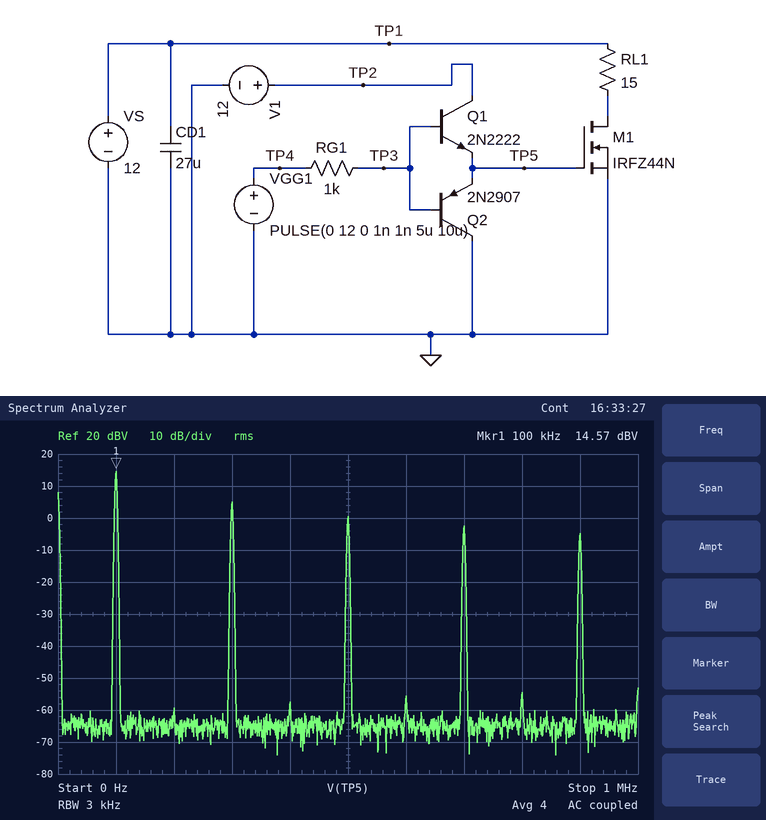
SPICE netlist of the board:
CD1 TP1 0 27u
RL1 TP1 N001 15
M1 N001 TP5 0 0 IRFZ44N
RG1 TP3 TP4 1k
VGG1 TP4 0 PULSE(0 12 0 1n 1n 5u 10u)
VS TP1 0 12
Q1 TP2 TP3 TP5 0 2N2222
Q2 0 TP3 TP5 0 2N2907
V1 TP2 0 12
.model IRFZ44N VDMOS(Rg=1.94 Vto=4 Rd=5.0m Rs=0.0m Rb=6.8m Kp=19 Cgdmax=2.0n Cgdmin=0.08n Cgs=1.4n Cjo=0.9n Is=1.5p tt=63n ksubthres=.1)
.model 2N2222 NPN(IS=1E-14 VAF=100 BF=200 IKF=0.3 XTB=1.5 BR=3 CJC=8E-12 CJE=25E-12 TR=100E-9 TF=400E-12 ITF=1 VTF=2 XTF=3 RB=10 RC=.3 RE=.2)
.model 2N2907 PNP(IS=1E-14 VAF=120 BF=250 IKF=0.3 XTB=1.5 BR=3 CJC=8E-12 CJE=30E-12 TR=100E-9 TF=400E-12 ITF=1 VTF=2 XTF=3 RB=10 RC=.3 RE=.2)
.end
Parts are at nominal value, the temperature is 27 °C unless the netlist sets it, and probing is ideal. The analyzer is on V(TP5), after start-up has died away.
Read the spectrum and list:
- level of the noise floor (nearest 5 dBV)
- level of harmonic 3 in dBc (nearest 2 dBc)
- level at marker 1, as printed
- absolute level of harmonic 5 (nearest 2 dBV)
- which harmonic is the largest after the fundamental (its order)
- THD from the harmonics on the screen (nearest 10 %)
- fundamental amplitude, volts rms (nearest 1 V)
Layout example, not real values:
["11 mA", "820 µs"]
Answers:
["-65 dBV", "-10 dBc", "14.57 dBV", "0 dBV", "3", "40 %", "5 V"]
